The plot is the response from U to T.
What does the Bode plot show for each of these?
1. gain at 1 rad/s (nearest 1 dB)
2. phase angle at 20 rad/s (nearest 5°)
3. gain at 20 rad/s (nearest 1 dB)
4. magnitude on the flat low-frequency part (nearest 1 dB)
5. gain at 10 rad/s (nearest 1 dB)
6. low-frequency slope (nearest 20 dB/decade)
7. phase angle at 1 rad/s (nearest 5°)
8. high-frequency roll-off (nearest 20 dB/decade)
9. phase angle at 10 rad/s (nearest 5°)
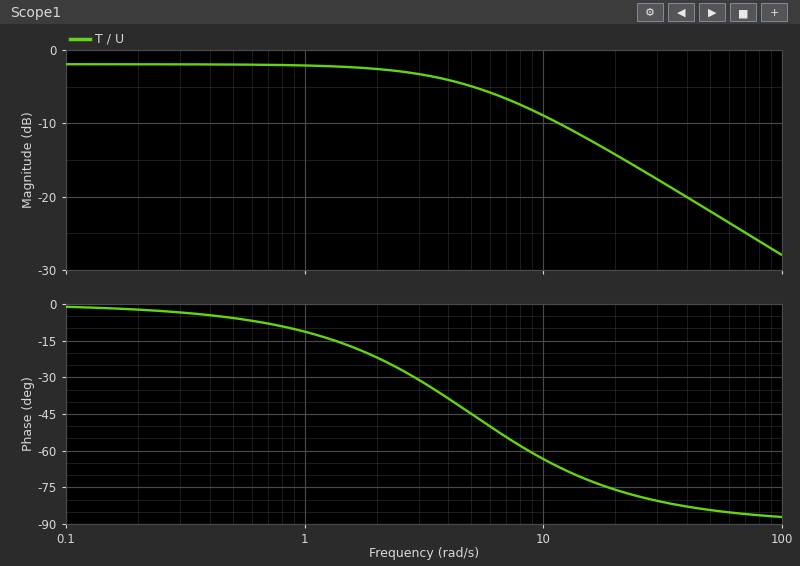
-2 dB
-75°
-14 dB
-2 dB
-9 dB
0 dB/decade
-10°
-20 dB/decade
-65°
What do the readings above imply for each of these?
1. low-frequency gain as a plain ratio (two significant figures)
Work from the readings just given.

0.79
